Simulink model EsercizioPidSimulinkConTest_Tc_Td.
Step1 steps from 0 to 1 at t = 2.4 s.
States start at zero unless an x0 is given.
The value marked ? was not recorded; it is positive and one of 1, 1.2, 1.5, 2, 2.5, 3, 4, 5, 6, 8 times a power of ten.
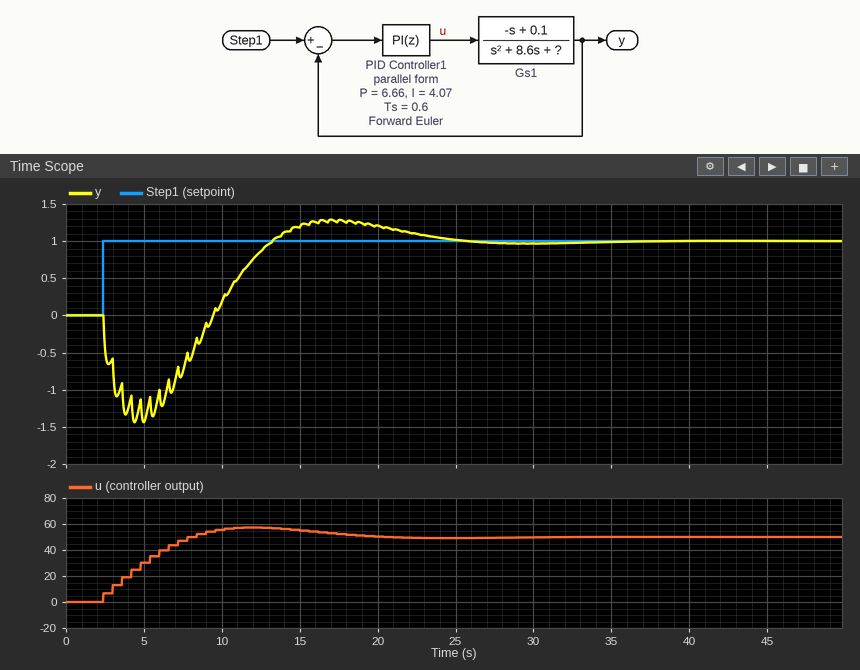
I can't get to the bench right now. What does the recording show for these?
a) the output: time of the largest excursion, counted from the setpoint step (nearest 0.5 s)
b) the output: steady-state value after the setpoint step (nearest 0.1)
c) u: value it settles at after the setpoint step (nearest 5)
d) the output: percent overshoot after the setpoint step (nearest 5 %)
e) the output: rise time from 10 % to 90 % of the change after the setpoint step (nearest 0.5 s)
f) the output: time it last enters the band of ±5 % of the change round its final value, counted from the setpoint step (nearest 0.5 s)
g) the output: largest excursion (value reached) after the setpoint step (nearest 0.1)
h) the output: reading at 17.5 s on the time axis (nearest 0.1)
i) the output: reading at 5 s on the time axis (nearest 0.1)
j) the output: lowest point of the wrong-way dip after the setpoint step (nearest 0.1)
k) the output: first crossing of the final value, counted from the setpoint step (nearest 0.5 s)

14.5 s
1.0
50
30 %
3.0 s
21.5 s
1.3
1.3
-1.4
-1.4
11.0 s
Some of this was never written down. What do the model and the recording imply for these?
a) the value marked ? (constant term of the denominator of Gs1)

5
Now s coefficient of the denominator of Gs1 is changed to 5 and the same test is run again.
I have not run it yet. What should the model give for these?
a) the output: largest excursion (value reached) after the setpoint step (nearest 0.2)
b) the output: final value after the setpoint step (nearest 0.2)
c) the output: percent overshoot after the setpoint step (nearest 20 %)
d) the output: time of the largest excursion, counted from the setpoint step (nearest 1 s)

1.4
1.0
40 %
7 s
